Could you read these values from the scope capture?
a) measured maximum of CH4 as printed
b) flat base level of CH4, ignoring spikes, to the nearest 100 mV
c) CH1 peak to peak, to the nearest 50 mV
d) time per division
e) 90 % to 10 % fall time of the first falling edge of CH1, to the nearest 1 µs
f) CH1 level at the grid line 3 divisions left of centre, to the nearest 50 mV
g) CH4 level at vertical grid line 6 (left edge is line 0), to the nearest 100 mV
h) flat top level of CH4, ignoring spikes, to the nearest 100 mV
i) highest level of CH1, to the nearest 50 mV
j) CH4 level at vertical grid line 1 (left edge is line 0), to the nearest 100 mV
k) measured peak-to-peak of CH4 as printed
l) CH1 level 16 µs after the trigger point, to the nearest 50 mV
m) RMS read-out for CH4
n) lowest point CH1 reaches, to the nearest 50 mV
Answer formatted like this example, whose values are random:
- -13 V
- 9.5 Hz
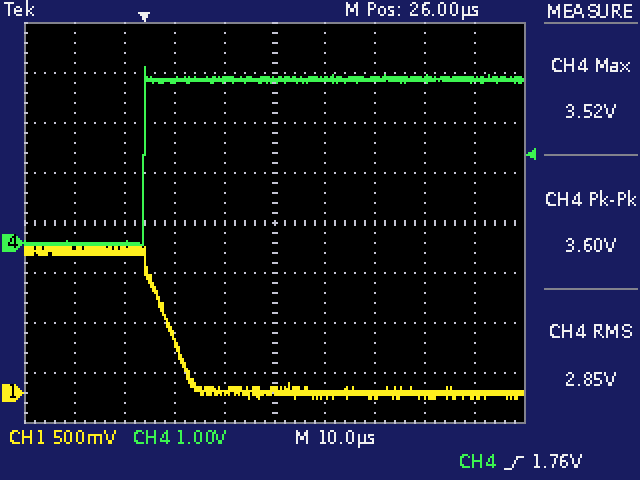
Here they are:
- 3.52 V
- 0.0 V
- 1.50 V
- 10 µs
- 9 µs
- 1.40 V
- 3.3 V
- 3.3 V
- 1.45 V
- 0.0 V
- 3.60 V
- 0 mV
- 2.85 V
- -50 mV
